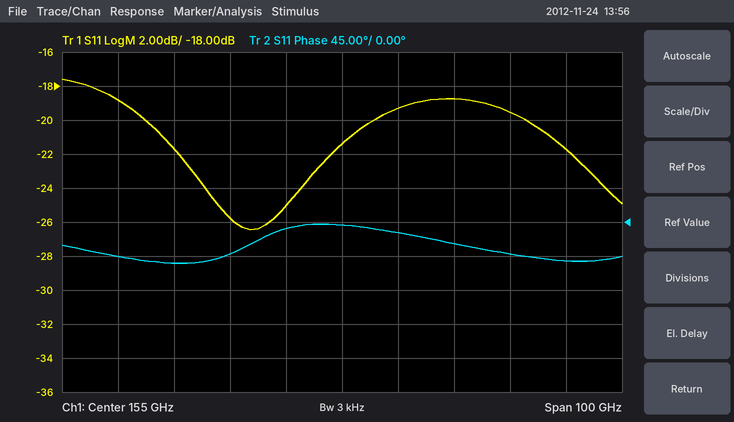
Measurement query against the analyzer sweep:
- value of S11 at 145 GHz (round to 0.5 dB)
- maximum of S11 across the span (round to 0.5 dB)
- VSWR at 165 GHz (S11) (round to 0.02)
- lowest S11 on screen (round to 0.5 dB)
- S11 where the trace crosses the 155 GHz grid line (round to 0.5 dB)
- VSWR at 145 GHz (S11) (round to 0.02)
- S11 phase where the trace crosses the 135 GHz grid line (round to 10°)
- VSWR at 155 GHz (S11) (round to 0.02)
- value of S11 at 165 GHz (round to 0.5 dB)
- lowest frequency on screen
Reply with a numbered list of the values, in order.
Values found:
1. -25.0 dB
2. -17.5 dB
3. 1.24
4. -26.5 dB
5. -21.5 dB
6. 1.12
7. -40°
8. 1.18
9. -19.5 dB
10. 105 GHz
